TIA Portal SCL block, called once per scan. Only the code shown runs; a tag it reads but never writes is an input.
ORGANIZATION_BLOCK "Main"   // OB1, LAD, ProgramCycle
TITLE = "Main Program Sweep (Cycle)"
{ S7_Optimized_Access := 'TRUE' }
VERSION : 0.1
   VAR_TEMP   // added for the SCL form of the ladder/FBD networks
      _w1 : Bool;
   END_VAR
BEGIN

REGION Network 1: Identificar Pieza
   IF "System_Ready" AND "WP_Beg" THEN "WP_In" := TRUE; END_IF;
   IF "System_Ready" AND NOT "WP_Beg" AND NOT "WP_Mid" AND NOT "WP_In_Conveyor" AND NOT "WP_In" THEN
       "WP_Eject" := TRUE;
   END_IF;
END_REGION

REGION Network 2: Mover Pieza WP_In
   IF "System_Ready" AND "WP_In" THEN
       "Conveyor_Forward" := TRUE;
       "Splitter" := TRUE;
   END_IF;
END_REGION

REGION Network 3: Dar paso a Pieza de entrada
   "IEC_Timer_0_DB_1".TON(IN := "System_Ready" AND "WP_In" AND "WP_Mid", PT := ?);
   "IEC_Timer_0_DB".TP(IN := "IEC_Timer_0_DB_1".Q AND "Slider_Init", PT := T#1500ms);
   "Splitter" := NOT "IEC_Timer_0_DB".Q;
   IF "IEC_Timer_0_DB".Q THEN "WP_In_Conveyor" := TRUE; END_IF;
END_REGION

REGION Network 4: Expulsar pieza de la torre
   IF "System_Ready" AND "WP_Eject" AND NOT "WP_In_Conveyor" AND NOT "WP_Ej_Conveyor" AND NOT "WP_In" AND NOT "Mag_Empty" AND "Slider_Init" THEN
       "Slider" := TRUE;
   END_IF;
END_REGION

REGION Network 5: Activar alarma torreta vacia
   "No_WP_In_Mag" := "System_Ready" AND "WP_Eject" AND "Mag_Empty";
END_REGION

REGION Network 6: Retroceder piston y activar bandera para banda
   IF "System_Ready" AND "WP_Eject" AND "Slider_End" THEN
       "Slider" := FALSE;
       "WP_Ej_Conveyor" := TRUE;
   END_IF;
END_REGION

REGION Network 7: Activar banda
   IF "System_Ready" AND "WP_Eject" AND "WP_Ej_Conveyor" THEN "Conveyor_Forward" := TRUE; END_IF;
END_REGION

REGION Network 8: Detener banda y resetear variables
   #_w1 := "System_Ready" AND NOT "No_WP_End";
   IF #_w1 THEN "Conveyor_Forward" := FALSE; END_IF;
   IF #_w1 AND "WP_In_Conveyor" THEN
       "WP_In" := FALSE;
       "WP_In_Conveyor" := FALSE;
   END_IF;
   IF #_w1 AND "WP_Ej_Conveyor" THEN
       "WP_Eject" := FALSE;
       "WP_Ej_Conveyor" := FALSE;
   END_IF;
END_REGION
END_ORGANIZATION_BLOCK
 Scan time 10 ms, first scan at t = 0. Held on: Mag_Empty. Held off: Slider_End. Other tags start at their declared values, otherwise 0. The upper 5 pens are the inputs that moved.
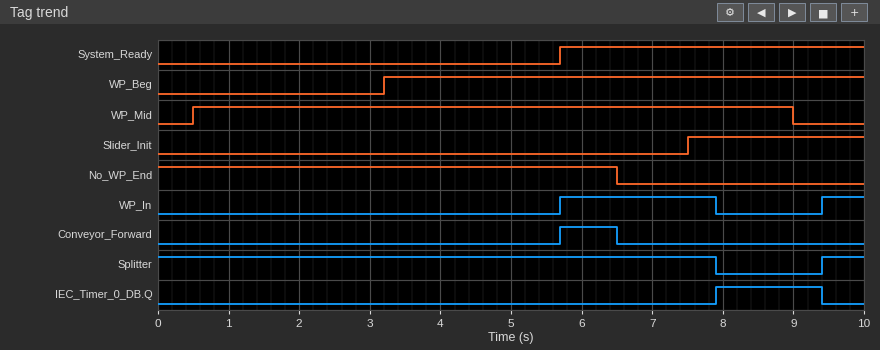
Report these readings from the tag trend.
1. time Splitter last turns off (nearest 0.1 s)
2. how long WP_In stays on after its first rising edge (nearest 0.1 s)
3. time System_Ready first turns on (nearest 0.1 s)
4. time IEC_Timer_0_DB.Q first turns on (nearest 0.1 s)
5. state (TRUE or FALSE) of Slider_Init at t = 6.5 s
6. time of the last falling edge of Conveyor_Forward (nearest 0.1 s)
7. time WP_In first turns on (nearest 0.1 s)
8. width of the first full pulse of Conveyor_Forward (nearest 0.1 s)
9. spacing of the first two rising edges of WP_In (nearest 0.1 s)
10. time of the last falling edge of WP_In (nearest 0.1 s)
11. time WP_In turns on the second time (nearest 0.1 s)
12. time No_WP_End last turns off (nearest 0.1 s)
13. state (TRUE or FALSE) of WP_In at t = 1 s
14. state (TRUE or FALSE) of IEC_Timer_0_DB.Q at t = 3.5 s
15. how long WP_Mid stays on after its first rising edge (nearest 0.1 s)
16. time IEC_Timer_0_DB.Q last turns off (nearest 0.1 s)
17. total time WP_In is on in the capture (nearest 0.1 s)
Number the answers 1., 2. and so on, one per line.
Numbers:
1. 7.9 s
2. 2.2 s
3. 5.7 s
4. 7.9 s
5. FALSE
6. 6.5 s
7. 5.7 s
8. 0.8 s
9. 3.7 s
10. 7.9 s
11. 9.4 s
12. 6.5 s
13. FALSE
14. FALSE
15. 8.5 s
16. 9.4 s
17. 2.8 s
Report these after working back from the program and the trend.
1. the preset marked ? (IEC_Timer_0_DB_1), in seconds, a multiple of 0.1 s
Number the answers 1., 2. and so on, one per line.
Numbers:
1. 2.2 s
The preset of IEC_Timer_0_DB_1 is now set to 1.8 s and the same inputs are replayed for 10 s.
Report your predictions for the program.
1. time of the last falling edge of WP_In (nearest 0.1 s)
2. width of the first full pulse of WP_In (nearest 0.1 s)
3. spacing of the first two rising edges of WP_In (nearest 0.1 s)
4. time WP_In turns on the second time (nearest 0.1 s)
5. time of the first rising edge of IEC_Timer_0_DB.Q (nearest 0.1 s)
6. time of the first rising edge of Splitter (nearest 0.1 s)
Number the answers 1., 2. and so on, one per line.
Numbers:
1. 7.5 s
2. 1.8 s
3. 3.3 s
4. 9.0 s
5. 7.5 s
6. 9.0 s
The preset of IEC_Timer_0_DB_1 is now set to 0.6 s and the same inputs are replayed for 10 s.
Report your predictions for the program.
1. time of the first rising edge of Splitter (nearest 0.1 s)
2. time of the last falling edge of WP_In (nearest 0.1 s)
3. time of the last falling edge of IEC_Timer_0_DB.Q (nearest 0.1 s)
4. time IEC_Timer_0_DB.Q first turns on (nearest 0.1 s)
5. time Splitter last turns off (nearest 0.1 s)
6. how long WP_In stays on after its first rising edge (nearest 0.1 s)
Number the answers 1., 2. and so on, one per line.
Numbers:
1. 9.0 s
2. 7.5 s
3. 9.0 s
4. 7.5 s
5. 7.5 s
6. 1.8 s
